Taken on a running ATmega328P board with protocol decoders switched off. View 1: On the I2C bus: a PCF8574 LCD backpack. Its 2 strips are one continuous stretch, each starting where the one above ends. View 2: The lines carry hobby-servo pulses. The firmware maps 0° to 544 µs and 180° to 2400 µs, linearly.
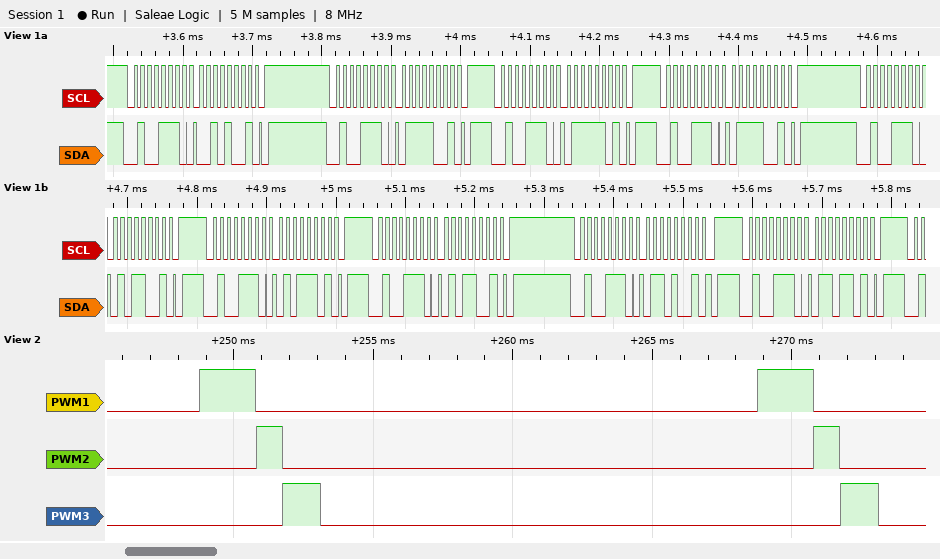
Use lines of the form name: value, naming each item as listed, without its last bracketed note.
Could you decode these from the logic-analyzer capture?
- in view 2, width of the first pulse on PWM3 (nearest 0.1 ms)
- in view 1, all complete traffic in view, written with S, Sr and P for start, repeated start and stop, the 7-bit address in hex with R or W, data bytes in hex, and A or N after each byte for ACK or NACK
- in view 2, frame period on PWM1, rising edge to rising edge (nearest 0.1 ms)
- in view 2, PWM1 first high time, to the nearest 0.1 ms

in view 2, width of the first pulse on PWM3: 1.4 ms
in view 1, all complete traffic in view, written with S, Sr and P for start, repeated start and stop, the 7-bit address in hex with R or W, data bytes in hex, and A or N after each byte for ACK or NACK: S 27W A 29 A P S 27W A 79 A P S 27W A 7D A P S 27W A 79 A P S 27W A 59 A P S 27W A 5D A P S 27W A 59 A P S 27W A 69 A P S 27W A 6D A P
in view 2, frame period on PWM1, rising edge to rising edge: 20.0 ms
in view 2, PWM1 first high time, to the nearest 0.1 ms: 2.0 ms
